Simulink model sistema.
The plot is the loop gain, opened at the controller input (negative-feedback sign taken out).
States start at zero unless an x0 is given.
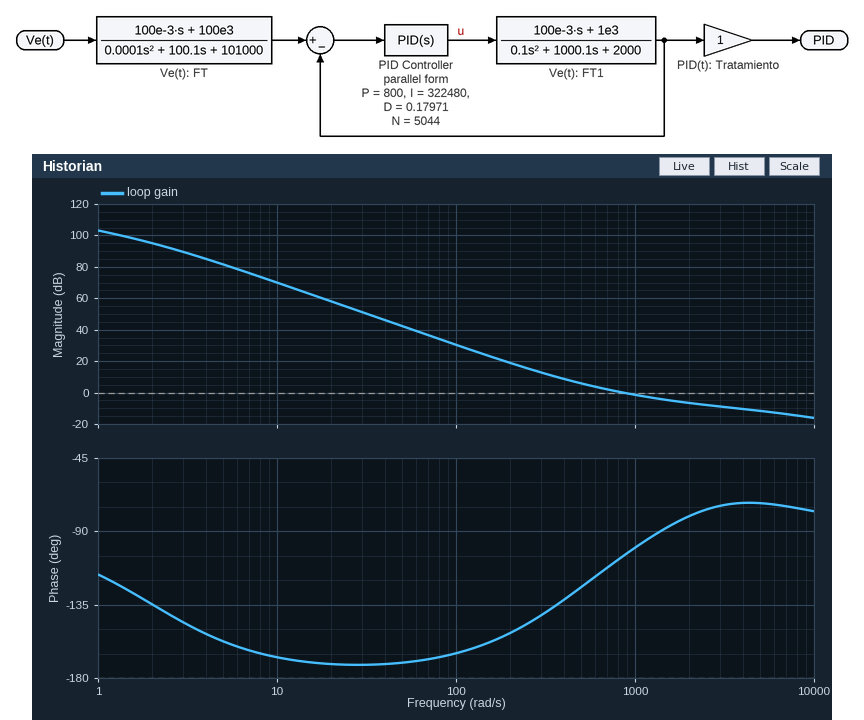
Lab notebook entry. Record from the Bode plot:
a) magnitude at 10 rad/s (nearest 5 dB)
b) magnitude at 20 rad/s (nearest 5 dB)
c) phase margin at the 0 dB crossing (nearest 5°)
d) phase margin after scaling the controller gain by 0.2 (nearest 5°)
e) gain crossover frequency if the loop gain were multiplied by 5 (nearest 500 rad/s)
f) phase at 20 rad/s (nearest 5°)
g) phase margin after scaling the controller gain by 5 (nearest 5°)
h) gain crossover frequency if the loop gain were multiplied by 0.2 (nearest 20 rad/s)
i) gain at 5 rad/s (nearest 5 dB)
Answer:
70 dB
60 dB
75°
35°
7500 rad/s
-170°
105°
280 rad/s
80 dB
